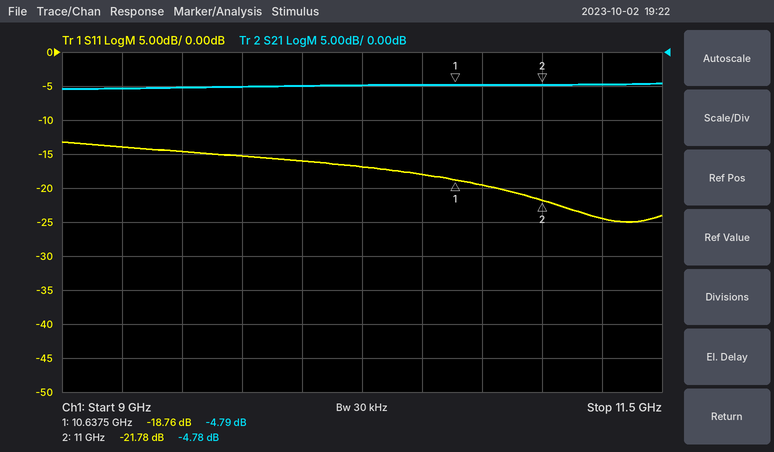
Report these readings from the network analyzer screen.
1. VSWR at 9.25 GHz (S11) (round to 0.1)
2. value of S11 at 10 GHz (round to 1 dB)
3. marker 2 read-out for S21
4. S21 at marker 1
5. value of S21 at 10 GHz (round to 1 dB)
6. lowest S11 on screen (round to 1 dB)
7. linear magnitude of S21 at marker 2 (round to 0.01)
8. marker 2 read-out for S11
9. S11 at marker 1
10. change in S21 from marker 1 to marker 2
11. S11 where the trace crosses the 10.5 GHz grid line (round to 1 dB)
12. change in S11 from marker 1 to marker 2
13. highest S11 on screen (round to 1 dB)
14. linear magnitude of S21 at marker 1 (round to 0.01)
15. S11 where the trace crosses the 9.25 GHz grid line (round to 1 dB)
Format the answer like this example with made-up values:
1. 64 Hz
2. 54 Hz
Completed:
1. 1.5
2. -16 dB
3. -4.78 dB
4. -4.79 dB
5. -5 dB
6. -25 dB
7. 0.58
8. -21.78 dB
9. -18.76 dB
10. 0.01 dB
11. -18 dB
12. -3.02 dB
13. -13 dB
14. 0.58
15. -14 dB
